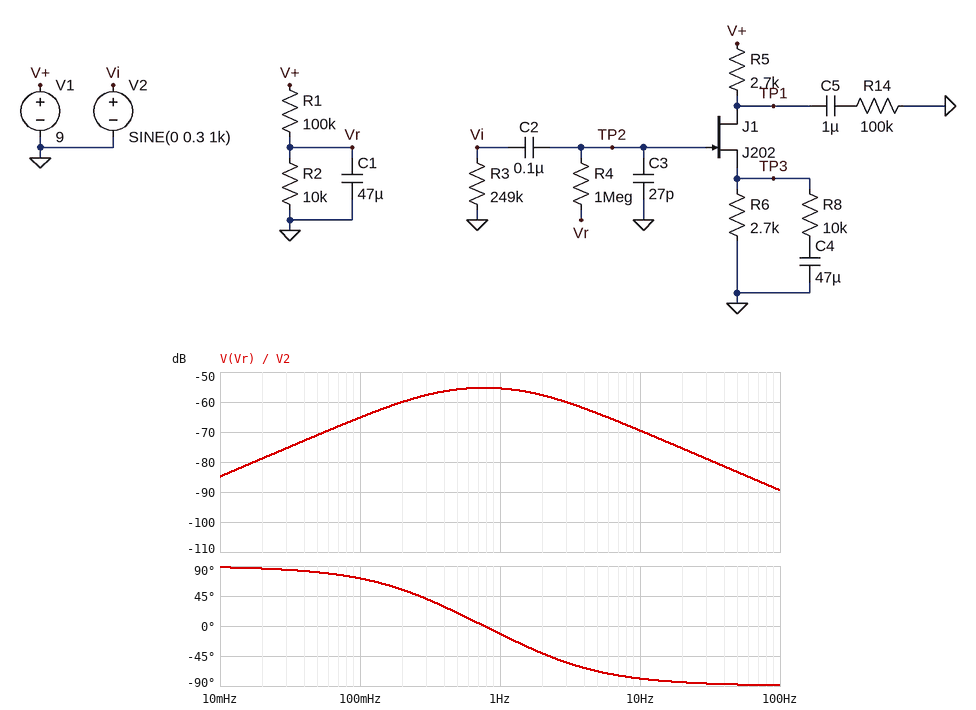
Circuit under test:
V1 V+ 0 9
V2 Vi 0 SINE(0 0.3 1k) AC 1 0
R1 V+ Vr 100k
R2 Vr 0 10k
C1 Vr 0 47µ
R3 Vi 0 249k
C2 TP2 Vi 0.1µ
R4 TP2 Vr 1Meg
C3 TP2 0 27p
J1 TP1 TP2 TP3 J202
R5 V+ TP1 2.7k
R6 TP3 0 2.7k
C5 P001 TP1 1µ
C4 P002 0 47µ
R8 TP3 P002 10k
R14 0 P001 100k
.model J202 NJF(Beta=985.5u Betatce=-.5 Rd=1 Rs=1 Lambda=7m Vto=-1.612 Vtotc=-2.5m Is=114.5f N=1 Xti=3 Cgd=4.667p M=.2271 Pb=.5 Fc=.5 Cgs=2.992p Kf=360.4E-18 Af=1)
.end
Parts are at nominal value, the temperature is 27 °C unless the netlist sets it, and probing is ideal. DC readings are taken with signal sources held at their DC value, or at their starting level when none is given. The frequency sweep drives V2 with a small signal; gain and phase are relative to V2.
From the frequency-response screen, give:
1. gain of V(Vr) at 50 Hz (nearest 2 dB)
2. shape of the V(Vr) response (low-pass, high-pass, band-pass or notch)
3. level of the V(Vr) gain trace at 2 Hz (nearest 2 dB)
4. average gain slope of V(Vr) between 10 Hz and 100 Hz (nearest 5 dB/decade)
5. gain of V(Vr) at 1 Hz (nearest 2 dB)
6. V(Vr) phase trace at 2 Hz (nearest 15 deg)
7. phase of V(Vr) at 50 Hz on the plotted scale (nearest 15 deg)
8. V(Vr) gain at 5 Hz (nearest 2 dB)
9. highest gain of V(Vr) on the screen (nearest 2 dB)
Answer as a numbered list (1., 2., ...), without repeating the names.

1. -84 dB
2. band-pass
3. -58 dB
4. -20 dB/decade
5. -56 dB
6. -45 deg
7. -90 deg
8. -64 dB
9. -56 dB
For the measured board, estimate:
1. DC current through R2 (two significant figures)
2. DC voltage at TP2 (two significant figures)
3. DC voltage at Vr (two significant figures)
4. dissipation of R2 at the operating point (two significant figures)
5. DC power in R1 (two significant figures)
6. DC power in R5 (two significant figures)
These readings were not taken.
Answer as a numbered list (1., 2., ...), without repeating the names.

1. 82 µA
2. 820 mV
3. 820 mV
4. 67 µW
5. 670 µW
6. 1.0 mW
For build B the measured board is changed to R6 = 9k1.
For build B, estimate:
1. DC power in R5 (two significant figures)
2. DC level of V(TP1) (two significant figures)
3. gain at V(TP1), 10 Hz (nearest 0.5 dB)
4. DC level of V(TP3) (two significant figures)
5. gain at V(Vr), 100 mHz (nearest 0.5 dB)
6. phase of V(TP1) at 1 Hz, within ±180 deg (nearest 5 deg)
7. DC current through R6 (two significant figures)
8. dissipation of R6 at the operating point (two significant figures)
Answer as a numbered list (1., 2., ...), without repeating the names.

1. 130 µW
2. 8.4 V
3. -7.0 dB
4. 2.0 V
5. -65.0 dB
6. -115 deg
7. 220 µA
8. 430 µW
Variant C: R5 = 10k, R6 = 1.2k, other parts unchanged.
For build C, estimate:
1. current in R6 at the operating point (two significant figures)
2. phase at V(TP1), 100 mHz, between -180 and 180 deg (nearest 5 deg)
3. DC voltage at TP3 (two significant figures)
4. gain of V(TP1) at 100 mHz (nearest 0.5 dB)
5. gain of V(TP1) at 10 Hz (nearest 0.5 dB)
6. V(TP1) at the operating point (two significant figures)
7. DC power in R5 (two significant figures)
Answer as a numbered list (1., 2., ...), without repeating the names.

1. 780 µA
2. -95 deg
3. 930 mV
4. -38.0 dB
5. -14.0 dB
6. 1.2 V
7. 6.0 mW
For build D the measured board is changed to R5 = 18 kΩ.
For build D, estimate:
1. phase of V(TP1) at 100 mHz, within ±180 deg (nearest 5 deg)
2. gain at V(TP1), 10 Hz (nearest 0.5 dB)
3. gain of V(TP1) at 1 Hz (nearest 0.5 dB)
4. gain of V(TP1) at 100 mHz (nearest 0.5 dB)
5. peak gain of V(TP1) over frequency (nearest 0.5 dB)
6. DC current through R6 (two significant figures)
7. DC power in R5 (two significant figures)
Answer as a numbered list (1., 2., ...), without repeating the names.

1. -95 deg
2. -17.5 dB
3. -22.5 dB
4. -41.0 dB
5. -17.0 dB
6. 430 µA
7. 3.3 mW
